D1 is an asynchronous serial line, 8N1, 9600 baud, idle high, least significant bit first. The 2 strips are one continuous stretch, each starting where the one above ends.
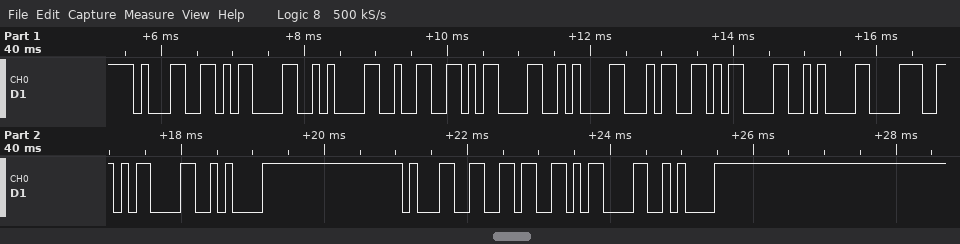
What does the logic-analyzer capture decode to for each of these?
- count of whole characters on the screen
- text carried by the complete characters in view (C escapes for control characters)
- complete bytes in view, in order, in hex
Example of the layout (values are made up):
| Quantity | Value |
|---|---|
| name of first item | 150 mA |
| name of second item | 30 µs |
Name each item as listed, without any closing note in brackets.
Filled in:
| Quantity | Value |
|---|---|
| count of whole characters on the screen | 16 |
| text carried by the complete characters in view | "1\r\n2\r\n4\r\n8\r\n16\r\n" |
| complete bytes in view, in order, in hex | 0x31 0x0D 0x0A 0x32 0x0D 0x0A 0x34 0x0D 0x0A 0x38 0x0D 0x0A 0x31 0x36 0x0D 0x0A |
